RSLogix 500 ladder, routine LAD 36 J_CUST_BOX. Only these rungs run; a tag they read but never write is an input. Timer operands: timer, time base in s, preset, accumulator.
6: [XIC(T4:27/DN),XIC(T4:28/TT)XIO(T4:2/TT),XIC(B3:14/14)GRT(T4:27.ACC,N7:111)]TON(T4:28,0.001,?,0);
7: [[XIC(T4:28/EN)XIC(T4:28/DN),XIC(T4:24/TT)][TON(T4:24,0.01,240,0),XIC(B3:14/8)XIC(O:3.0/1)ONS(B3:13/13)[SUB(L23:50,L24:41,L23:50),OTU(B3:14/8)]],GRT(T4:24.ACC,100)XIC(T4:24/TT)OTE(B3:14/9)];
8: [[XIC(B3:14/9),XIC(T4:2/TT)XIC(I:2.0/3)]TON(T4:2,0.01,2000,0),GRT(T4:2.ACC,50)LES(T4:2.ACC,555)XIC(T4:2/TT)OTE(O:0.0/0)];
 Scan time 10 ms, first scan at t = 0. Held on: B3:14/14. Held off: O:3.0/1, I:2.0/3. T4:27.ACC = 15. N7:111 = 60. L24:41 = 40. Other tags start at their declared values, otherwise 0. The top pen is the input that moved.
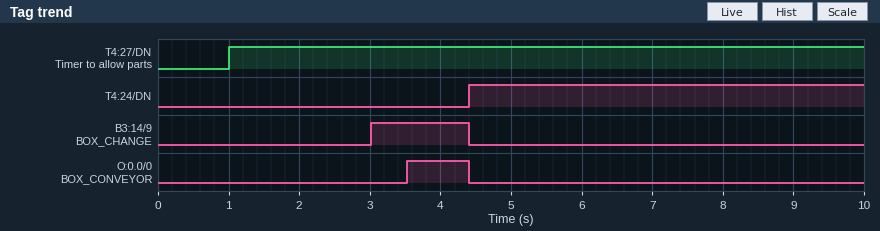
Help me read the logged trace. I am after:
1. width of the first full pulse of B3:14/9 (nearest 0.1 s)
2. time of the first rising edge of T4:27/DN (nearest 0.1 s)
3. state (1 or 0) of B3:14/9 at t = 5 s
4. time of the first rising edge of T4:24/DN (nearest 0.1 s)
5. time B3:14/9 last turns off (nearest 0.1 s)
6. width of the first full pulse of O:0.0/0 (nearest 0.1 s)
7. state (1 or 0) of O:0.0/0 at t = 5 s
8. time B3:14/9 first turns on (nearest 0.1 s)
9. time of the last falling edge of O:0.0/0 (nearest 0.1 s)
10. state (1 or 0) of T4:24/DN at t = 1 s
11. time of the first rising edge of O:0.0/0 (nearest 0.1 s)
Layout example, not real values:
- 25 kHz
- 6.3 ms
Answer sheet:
- 1.4 s
- 1.0 s
- 0
- 4.4 s
- 4.4 s
- 0.9 s
- 0
- 3.0 s
- 4.4 s
- 0
- 3.5 s
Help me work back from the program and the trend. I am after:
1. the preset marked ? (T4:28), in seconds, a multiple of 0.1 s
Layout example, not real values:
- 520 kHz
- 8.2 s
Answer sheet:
- 1.0 s
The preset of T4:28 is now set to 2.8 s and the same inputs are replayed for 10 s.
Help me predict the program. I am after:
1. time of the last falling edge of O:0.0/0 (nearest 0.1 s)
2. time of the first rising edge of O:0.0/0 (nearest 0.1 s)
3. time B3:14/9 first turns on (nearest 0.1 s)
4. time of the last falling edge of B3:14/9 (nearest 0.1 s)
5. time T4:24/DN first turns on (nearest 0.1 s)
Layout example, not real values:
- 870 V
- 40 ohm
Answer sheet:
- 6.2 s
- 5.3 s
- 4.8 s
- 6.2 s
- 6.2 s
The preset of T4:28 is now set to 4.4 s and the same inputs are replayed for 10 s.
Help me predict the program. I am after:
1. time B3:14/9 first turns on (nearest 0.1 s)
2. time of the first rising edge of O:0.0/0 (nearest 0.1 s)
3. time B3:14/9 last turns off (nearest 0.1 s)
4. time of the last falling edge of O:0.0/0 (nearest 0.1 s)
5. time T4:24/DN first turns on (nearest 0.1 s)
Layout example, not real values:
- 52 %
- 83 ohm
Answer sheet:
- 6.4 s
- 6.9 s
- 7.8 s
- 7.8 s
- 7.8 s
